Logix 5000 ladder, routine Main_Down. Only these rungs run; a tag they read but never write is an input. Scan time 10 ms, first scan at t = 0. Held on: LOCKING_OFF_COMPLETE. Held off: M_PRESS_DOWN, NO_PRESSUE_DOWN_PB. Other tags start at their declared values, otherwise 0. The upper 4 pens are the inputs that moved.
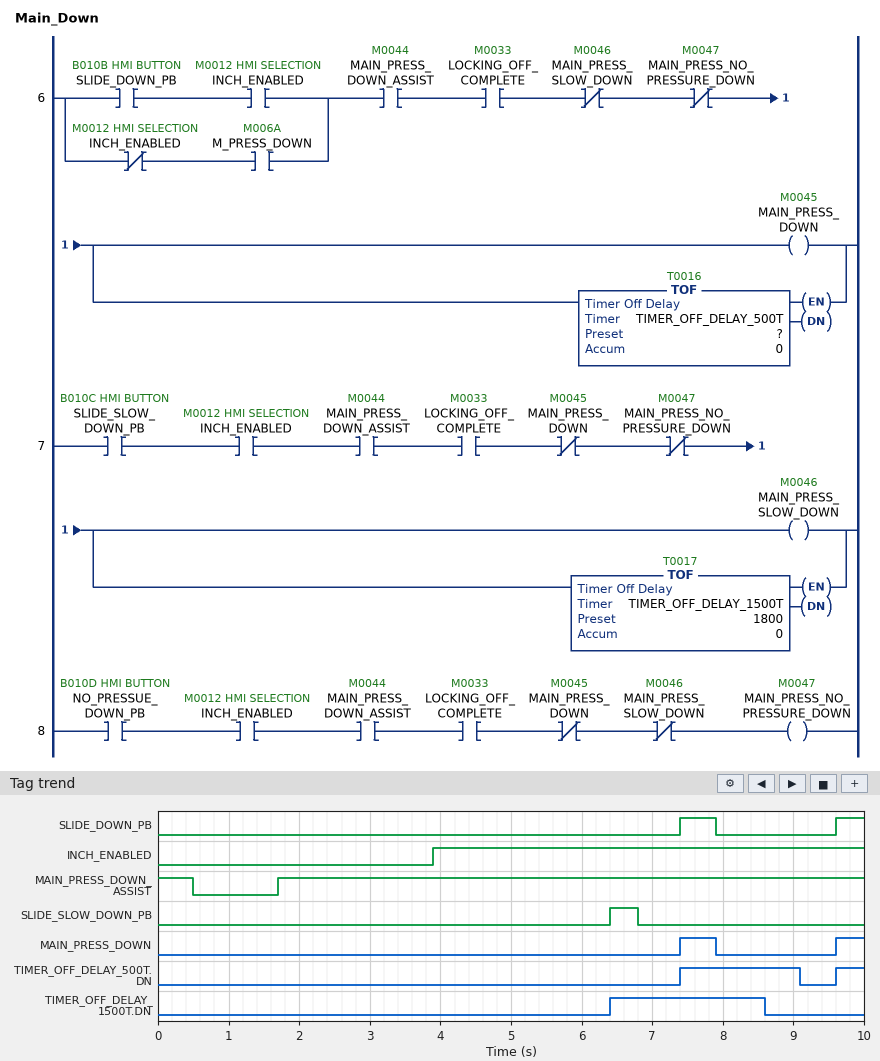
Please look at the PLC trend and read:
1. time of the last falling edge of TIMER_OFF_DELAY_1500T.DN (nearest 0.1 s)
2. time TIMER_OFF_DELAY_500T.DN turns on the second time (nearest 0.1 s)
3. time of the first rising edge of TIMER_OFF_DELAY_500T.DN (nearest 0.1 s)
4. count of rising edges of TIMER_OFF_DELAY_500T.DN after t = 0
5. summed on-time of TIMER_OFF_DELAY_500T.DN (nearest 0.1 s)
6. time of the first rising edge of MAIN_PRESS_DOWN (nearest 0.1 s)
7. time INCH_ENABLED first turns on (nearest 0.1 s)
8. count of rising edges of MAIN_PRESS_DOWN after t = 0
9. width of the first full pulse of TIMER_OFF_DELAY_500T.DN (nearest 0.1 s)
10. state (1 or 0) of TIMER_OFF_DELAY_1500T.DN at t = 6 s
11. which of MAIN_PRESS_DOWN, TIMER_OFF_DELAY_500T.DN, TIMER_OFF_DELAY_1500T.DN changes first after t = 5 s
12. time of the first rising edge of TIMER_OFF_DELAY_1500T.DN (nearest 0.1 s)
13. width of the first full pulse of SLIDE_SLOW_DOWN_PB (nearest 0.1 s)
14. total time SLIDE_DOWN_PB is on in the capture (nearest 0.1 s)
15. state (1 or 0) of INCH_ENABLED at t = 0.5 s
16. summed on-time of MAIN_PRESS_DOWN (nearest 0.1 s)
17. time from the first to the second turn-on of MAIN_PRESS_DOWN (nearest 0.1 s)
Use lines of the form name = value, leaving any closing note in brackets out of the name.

time of the last falling edge of TIMER_OFF_DELAY_1500T.DN = 8.6 s
time TIMER_OFF_DELAY_500T.DN turns on the second time = 9.6 s
time of the first rising edge of TIMER_OFF_DELAY_500T.DN = 7.4 s
count of rising edges of TIMER_OFF_DELAY_500T.DN after t = 0 = 2
summed on-time of TIMER_OFF_DELAY_500T.DN = 2.1 s
time of the first rising edge of MAIN_PRESS_DOWN = 7.4 s
time INCH_ENABLED first turns on = 3.9 s
count of rising edges of MAIN_PRESS_DOWN after t = 0 = 2
width of the first full pulse of TIMER_OFF_DELAY_500T.DN = 1.7 s
state (1 or 0) of TIMER_OFF_DELAY_1500T.DN at t = 6 s = 0
which of MAIN_PRESS_DOWN, TIMER_OFF_DELAY_500T.DN, TIMER_OFF_DELAY_1500T.DN changes first after t = 5 s = TIMER_OFF_DELAY_1500T.DN
time of the first rising edge of TIMER_OFF_DELAY_1500T.DN = 6.4 s
width of the first full pulse of SLIDE_SLOW_DOWN_PB = 0.4 s
total time SLIDE_DOWN_PB is on in the capture = 0.9 s
state (1 or 0) of INCH_ENABLED at t = 0.5 s = 0
summed on-time of MAIN_PRESS_DOWN = 0.9 s
time from the first to the second turn-on of MAIN_PRESS_DOWN = 2.2 s
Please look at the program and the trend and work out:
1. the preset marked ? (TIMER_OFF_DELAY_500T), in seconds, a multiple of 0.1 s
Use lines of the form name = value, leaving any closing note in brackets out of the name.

the preset marked ? (TIMER_OFF_DELAY_500T), in seconds, a multiple of 0.1 s = 1.2 s
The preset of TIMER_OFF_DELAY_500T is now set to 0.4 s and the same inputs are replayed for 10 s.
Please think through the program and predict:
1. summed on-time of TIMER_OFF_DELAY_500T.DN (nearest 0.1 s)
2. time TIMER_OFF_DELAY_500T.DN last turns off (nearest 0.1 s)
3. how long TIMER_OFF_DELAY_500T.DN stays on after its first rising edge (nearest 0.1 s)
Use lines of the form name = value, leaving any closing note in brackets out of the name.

summed on-time of TIMER_OFF_DELAY_500T.DN = 1.3 s
time TIMER_OFF_DELAY_500T.DN last turns off = 8.3 s
how long TIMER_OFF_DELAY_500T.DN stays on after its first rising edge = 0.9 s
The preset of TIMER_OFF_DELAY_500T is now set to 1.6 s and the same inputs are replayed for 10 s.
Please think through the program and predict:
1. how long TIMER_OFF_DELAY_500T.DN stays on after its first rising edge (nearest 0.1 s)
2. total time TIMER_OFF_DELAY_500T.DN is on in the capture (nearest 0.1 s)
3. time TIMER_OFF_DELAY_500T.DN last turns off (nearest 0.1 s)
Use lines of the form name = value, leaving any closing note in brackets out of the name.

how long TIMER_OFF_DELAY_500T.DN stays on after its first rising edge = 2.1 s
total time TIMER_OFF_DELAY_500T.DN is on in the capture = 2.5 s
time TIMER_OFF_DELAY_500T.DN last turns off = 9.5 s
